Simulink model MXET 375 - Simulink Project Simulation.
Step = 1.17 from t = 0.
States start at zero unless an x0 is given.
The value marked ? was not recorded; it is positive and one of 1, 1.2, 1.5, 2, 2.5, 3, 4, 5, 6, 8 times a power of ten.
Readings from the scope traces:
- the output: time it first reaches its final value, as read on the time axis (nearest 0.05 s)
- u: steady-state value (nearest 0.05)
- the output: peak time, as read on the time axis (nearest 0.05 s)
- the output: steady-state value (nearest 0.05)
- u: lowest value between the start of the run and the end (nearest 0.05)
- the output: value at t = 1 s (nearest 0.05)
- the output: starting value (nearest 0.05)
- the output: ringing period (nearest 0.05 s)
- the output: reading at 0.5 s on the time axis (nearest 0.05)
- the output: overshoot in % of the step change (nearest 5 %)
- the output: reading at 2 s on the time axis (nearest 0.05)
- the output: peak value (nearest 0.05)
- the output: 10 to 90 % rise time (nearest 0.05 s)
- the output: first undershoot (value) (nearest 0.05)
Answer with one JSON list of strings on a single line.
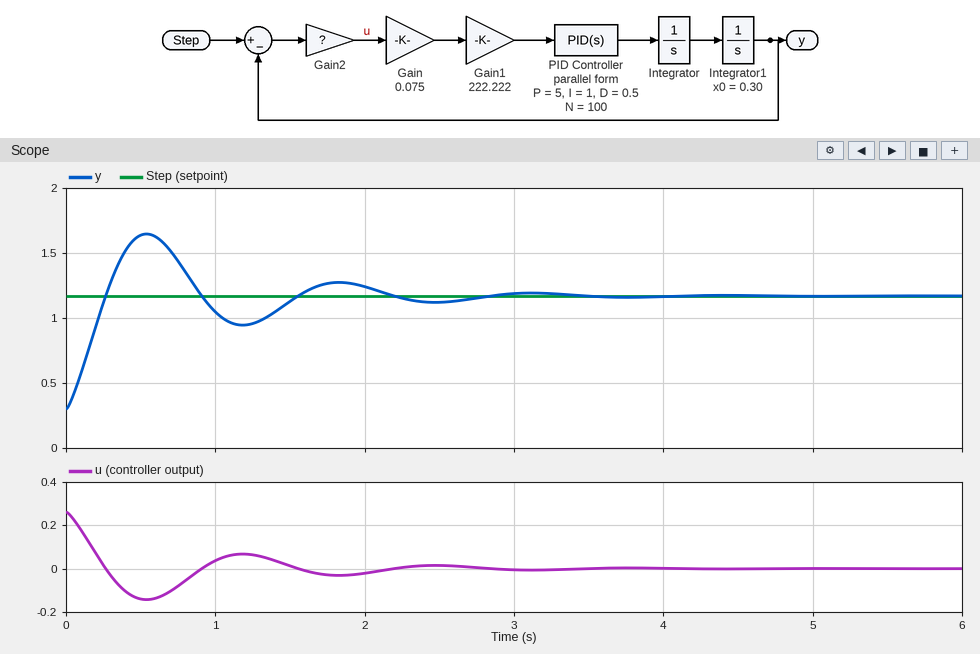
["0.25 s", "0.00", "0.55 s", "1.15", "-0.15", "1.05", "0.30", "1.30 s", "1.65", "55 %", "1.25", "1.65", "0.20 s", "0.95"]
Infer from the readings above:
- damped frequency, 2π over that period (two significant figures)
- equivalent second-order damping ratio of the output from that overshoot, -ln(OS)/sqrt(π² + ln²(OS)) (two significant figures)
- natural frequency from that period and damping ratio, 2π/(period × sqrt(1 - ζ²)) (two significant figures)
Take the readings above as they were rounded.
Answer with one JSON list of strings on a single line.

["4.8 rad/s", "0.19", "4.9 rad/s"]
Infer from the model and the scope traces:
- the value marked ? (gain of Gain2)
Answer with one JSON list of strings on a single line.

["0.3"]
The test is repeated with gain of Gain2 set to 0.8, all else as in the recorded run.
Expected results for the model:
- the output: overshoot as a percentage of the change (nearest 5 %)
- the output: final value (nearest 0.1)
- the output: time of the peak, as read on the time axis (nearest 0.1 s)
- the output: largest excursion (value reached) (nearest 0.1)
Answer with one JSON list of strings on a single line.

["40 %", "1.2", "0.3 s", "1.5"]
